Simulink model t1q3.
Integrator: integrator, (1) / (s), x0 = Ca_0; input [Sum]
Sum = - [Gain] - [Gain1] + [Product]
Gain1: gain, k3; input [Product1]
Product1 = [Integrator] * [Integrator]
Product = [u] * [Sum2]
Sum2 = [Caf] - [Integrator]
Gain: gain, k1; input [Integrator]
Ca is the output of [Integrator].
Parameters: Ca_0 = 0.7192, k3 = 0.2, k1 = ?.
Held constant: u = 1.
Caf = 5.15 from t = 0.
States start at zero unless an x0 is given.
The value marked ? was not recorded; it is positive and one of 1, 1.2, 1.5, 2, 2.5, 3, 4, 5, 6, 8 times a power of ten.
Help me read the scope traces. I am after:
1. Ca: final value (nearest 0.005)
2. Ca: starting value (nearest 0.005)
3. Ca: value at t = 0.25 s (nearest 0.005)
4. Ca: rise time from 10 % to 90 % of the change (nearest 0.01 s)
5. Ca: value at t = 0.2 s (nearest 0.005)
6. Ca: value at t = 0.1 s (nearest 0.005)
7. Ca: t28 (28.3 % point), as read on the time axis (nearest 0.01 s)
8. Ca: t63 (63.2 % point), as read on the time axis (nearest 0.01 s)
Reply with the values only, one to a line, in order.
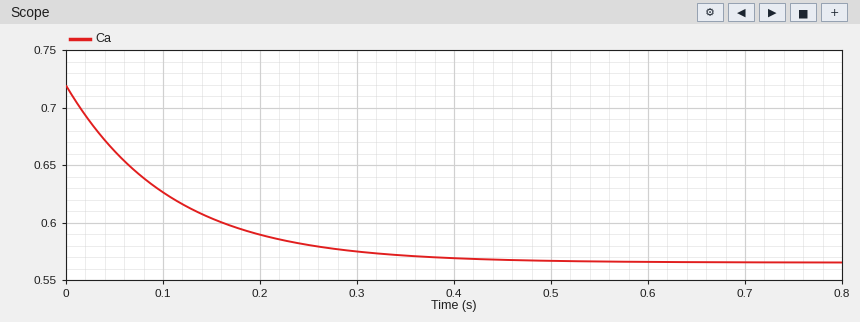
0.565
0.720
0.580
0.24 s
0.590
0.625
0.04 s
0.11 s
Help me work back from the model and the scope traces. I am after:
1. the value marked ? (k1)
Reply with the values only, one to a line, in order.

8
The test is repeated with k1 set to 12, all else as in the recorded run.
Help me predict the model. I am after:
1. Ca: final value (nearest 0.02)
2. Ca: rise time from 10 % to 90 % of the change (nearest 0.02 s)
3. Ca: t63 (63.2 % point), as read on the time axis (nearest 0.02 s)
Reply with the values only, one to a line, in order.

0.40
0.16 s
0.08 s
